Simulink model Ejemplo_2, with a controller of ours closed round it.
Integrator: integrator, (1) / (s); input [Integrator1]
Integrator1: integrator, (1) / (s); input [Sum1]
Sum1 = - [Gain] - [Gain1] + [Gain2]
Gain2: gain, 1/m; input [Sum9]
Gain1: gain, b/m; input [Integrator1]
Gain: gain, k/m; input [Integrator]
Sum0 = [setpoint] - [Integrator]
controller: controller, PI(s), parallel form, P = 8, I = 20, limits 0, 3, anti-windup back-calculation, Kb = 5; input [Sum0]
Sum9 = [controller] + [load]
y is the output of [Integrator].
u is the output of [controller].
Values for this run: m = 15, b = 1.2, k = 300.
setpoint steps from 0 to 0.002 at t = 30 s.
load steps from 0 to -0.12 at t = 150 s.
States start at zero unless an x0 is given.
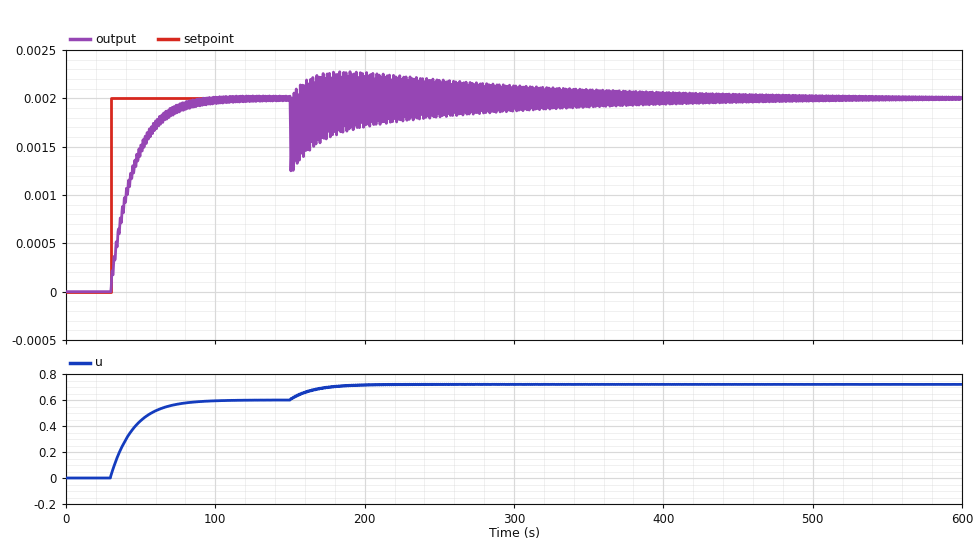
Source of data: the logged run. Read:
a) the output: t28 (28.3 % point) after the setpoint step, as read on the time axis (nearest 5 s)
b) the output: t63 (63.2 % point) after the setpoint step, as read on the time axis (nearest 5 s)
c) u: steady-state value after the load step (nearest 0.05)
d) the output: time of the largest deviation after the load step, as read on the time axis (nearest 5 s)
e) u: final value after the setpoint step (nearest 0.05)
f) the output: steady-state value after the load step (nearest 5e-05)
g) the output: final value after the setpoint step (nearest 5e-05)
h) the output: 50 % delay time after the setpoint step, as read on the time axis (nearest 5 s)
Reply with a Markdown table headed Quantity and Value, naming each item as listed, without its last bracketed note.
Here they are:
| Quantity | Value |
|---|---|
| the output: t28 (28.3 % point) after the setpoint step, as read on the time axis | 35 s |
| the output: t63 (63.2 % point) after the setpoint step, as read on the time axis | 45 s |
| u: steady-state value after the load step | 0.70 |
| the output: time of the largest deviation after the load step, as read on the time axis | 150 s |
| u: final value after the setpoint step | 0.60 |
| the output: steady-state value after the load step | 0.00200 |
| the output: final value after the setpoint step | 0.00200 |
| the output: 50 % delay time after the setpoint step, as read on the time axis | 40 s |
